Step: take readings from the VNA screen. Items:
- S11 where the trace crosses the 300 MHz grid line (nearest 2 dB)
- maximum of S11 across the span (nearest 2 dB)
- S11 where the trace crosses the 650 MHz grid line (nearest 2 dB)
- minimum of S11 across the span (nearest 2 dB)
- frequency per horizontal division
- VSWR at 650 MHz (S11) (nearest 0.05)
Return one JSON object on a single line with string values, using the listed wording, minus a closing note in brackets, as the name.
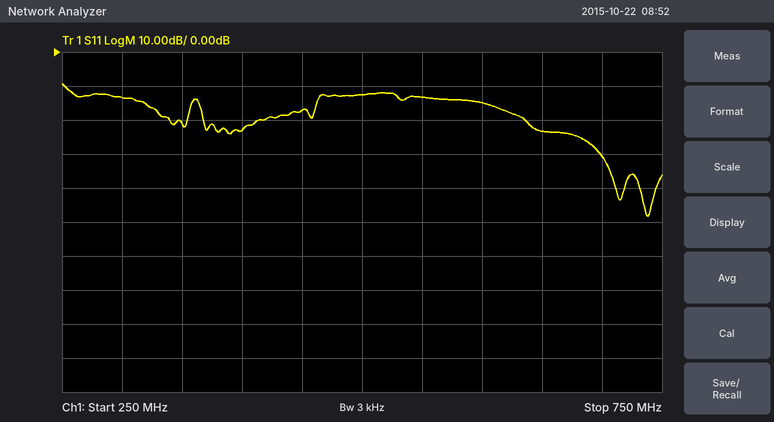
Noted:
{"S11 where the trace crosses the 300 MHz grid line": "-14 dB", "maximum of S11 across the span": "-10 dB", "S11 where the trace crosses the 650 MHz grid line": "-24 dB", "minimum of S11 across the span": "-48 dB", "frequency per horizontal division": "50 MHz", "VSWR at 650 MHz (S11)": "1.15"}
